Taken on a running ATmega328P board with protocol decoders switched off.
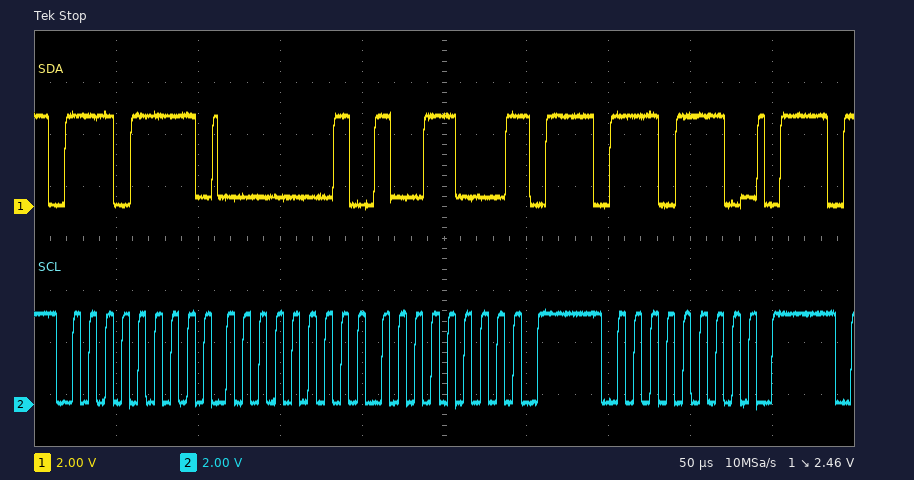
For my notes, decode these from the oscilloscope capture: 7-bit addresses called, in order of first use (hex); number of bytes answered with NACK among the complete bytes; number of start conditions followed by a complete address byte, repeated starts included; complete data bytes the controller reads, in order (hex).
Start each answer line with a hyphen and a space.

- 0x77
- 1
- 2
- 01 98
